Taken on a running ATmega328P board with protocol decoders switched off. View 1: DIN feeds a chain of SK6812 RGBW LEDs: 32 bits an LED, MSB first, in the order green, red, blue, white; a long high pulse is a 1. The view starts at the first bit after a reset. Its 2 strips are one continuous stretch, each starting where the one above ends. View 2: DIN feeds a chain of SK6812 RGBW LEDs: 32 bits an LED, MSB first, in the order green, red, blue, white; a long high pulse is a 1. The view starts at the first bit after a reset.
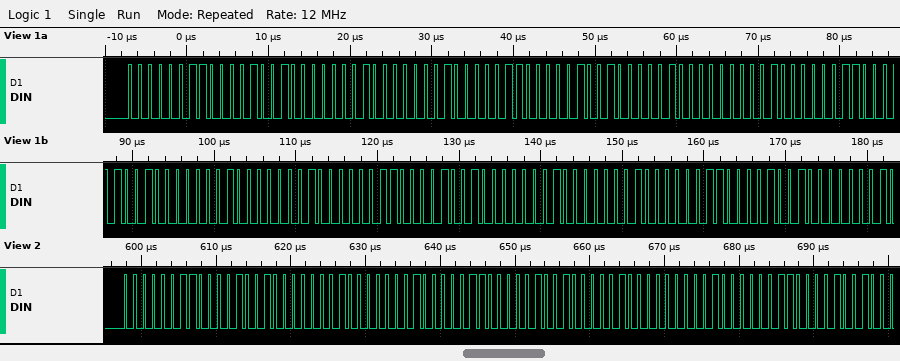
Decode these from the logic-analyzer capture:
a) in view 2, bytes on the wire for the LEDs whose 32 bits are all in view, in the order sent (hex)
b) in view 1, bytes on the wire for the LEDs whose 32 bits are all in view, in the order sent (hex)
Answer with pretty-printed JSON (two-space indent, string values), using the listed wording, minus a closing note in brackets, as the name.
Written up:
{
  "in view 2, bytes on the wire for the LEDs whose 32 bits are all in view, in the order sent": "03 09 01 01 06 09 04 01",
  "in view 1, bytes on the wire for the LEDs whose 32 bits are all in view, in the order sent": "03 09 01 01 06 09 04 01 03 09 01 01 03 09 01 01"
}
